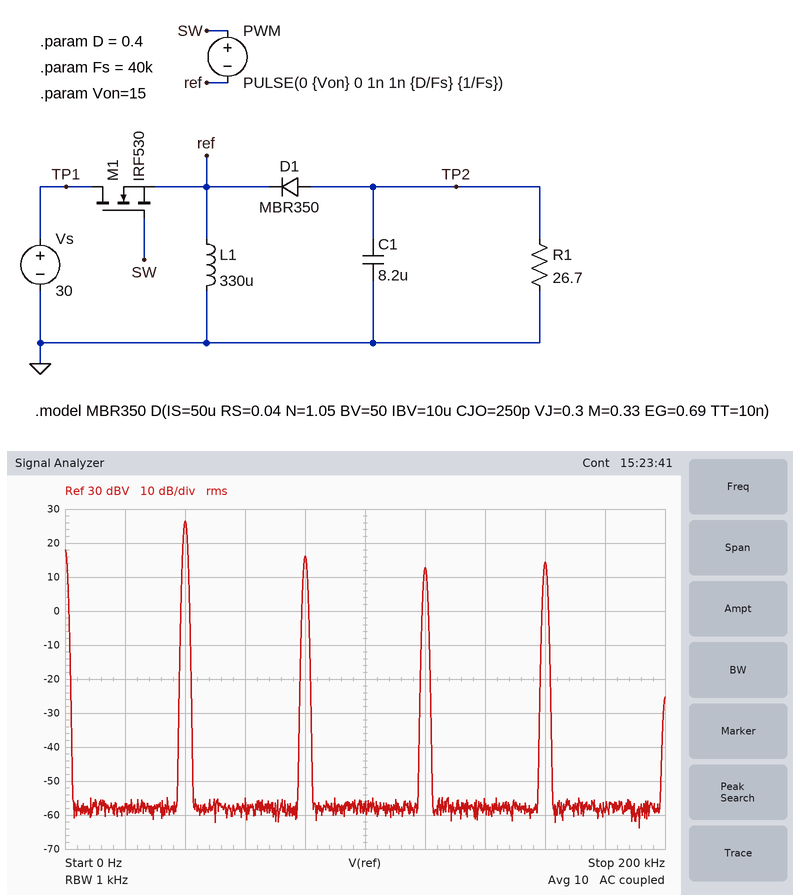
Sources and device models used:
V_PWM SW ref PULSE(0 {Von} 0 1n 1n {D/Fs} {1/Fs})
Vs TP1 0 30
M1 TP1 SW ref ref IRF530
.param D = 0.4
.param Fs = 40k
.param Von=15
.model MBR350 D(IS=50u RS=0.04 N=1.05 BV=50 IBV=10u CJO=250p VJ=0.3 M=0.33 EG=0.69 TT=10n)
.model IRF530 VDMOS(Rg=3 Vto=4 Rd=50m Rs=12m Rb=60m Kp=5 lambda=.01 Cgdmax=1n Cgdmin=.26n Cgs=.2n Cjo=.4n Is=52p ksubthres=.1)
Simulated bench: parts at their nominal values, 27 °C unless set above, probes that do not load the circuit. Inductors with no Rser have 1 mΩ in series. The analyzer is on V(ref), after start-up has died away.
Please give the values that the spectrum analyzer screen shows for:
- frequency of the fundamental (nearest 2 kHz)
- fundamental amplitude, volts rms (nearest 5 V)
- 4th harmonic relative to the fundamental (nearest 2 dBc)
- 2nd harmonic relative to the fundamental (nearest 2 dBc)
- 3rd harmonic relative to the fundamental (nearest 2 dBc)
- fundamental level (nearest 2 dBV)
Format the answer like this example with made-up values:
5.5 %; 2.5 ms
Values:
40 kHz; 20 V; -12 dBc; -10 dBc; -14 dBc; 26 dBV
